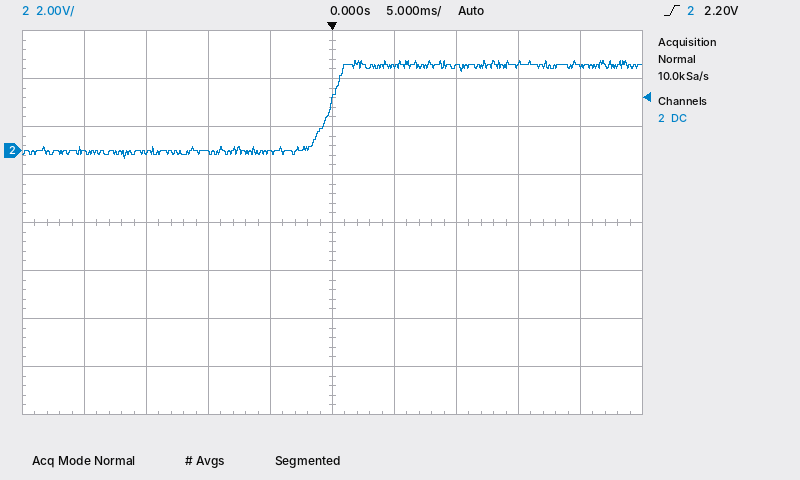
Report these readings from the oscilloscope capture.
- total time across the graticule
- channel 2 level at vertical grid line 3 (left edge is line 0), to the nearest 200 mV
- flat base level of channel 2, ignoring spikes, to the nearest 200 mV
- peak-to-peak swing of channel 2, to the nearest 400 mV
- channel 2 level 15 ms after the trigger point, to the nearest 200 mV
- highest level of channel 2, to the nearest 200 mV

50 ms
0.0 V
0.0 V
4.0 V
3.6 V
3.8 V
